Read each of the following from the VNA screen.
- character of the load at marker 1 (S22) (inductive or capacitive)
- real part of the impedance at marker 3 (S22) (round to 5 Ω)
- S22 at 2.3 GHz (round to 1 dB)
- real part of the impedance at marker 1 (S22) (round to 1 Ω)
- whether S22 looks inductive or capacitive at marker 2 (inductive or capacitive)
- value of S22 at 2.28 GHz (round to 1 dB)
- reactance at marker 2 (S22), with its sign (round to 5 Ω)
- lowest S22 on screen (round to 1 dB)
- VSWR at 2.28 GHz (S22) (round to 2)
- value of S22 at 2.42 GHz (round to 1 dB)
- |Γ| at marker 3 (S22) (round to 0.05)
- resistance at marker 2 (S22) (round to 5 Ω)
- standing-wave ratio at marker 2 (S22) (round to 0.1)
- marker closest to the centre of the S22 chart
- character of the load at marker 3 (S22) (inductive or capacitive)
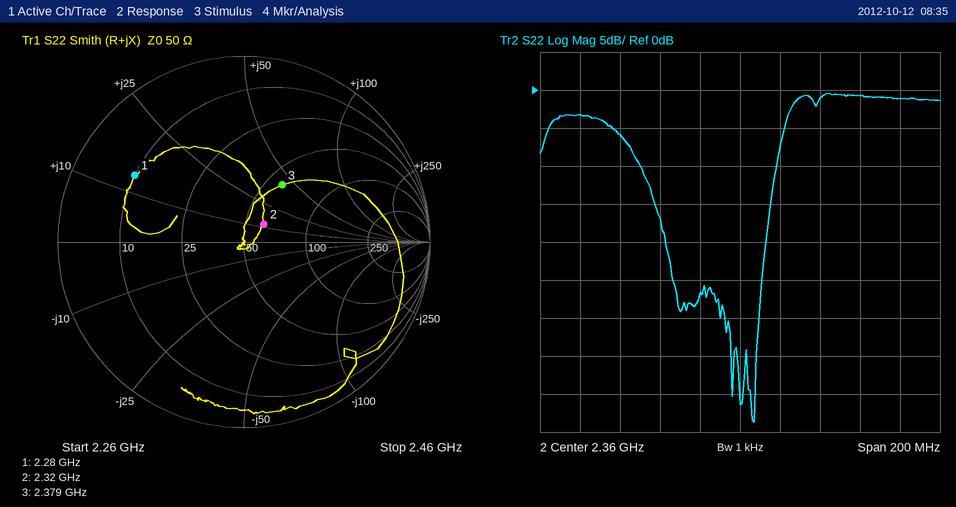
inductive
60 Ω
-6 dB
10 Ω
inductive
-3 dB
+10 Ω
-44 dB
6
-1 dB
0.35
60 Ω
1.3
marker 2
inductive
